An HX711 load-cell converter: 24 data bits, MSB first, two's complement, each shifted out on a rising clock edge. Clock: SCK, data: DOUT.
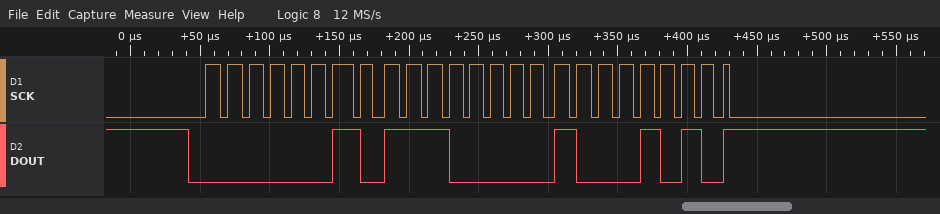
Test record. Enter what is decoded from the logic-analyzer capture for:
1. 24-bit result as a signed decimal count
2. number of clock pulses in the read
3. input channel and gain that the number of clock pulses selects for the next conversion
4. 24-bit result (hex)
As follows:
188554
25
channel A, gain 128
0x02E08A
